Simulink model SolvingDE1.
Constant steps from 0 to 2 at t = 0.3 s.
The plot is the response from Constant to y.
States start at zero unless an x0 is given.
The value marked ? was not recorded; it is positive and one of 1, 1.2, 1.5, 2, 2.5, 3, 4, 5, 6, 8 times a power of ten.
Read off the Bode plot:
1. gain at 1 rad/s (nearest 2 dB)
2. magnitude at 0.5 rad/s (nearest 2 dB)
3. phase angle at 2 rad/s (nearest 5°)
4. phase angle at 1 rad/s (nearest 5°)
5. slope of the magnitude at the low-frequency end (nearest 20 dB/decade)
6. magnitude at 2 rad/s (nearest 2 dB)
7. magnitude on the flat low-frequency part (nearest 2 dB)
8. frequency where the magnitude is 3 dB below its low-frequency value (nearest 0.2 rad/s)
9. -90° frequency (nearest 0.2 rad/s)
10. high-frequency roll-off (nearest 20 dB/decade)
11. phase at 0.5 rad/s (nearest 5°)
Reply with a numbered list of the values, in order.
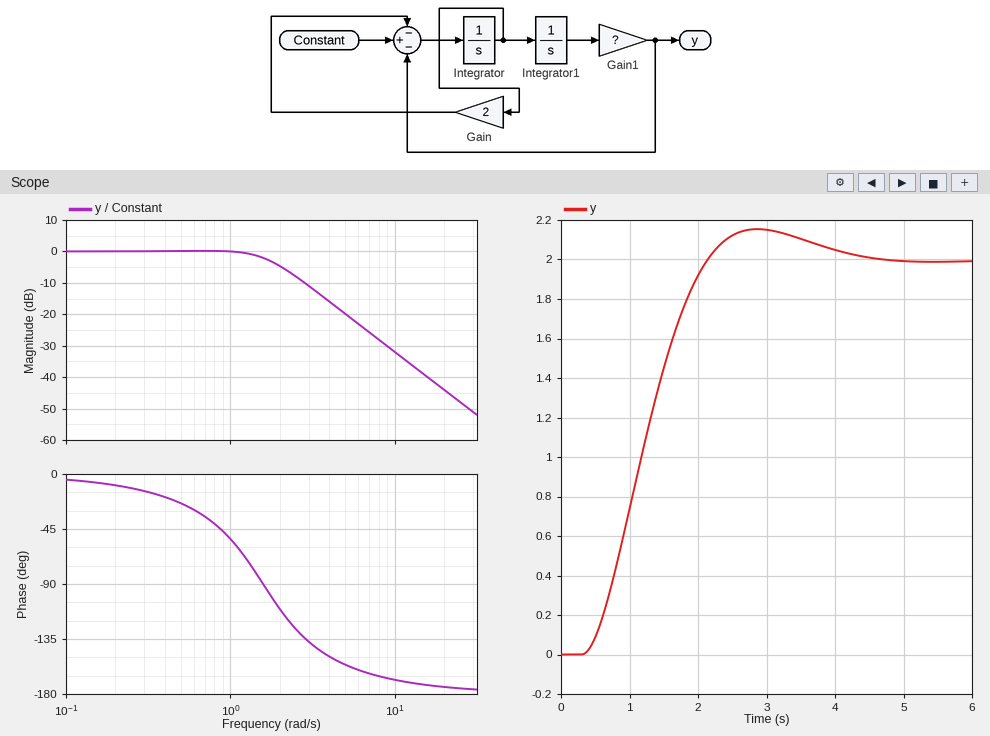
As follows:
1. 0 dB
2. 0 dB
3. -110°
4. -55°
5. 0 dB/decade
6. -4 dB
7. 0 dB
8. 1.8 rad/s
9. 1.6 rad/s
10. -40 dB/decade
11. -25°
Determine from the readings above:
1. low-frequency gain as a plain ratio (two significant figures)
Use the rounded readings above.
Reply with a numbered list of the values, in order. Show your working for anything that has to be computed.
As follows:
1. 10^(0 / 20) = 1.0
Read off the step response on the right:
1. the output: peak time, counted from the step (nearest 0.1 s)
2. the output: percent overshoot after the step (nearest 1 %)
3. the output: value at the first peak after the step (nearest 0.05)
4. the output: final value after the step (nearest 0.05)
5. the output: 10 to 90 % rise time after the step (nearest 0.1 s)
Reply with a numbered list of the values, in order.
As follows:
1. 2.6 s
2. 8 %
3. 2.15
4. 2.00
5. 1.2 s
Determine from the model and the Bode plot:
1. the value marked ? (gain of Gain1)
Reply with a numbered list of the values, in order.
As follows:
1. 2.5
